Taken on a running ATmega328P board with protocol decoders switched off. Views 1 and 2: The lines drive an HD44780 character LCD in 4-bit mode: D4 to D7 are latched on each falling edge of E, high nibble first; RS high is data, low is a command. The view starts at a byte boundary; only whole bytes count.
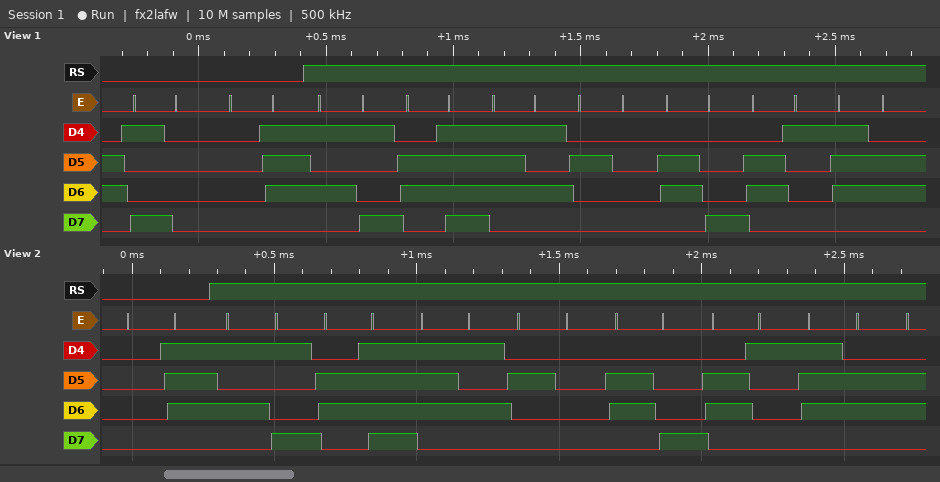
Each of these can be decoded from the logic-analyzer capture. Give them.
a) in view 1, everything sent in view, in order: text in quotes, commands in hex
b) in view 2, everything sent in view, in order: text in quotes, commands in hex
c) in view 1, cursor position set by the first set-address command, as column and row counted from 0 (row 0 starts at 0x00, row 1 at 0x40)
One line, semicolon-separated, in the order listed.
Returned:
0x90 0x07 "You hav"; 0x07 "You hav"; column 16, row 0
